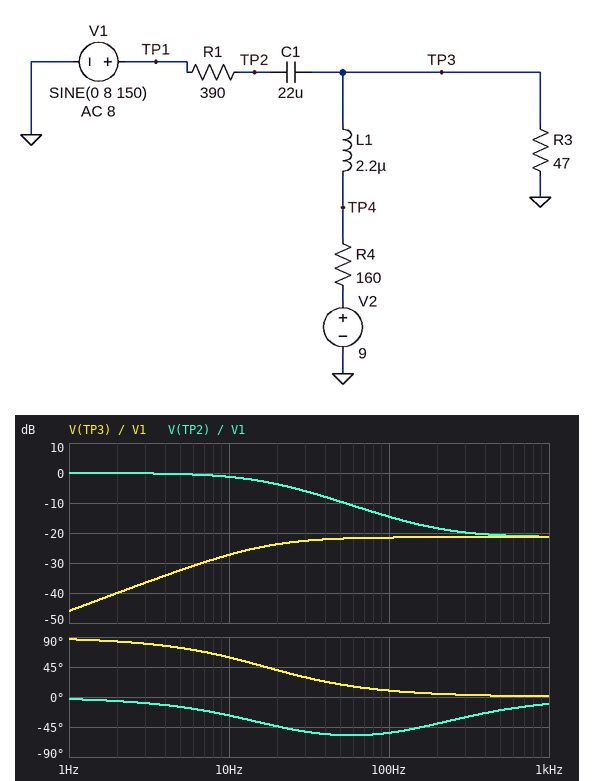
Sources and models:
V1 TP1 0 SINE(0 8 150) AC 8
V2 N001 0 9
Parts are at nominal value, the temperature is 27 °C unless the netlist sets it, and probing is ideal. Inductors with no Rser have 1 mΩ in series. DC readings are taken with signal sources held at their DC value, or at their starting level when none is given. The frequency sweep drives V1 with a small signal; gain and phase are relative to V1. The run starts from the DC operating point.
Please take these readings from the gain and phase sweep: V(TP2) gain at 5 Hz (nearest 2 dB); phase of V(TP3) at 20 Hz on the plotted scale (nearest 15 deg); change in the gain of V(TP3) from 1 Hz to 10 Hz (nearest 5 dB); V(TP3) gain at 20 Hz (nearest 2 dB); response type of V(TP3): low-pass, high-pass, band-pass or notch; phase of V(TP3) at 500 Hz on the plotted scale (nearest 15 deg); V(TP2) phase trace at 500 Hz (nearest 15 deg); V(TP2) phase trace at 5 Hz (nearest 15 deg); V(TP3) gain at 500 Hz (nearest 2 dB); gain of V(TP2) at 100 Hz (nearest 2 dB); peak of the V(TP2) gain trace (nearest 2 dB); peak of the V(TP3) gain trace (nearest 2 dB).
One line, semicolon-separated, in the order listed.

0 dB; 45 deg; 20 dB; -24 dB; high-pass; 0 deg; -15 deg; -15 deg; -22 dB; -14 dB; 0 dB; -22 dB
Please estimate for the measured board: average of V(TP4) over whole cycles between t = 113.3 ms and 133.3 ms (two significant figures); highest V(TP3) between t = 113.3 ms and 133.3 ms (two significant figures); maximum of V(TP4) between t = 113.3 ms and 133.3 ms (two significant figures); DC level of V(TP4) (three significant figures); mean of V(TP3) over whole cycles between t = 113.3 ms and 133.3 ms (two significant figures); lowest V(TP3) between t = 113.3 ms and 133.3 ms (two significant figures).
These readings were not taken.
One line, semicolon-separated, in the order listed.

2.0 V; 2.7 V; 2.7 V; 2.04 V; 2.0 V; 1.4 V
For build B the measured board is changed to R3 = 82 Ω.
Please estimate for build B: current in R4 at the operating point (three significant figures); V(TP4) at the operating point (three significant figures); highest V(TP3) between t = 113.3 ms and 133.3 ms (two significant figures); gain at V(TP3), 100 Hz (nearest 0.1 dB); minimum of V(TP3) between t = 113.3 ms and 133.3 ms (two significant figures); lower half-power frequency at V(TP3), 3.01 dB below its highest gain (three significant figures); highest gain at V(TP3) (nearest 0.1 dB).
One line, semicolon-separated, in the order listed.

37.2 mA; 3.05 V; 4.0 V; -18.4 dB; 2.1 V; 16.3 Hz; -18.3 dB
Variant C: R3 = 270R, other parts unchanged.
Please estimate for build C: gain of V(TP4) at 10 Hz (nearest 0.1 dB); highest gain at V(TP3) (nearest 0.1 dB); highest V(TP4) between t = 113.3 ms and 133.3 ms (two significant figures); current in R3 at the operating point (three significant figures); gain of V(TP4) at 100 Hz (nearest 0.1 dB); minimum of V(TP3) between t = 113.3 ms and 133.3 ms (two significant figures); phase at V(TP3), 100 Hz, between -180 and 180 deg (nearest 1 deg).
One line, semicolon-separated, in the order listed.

-18.8 dB; -13.8 dB; 7.3 V; 20.9 mA; -13.9 dB; 4.0 V; 8 deg
